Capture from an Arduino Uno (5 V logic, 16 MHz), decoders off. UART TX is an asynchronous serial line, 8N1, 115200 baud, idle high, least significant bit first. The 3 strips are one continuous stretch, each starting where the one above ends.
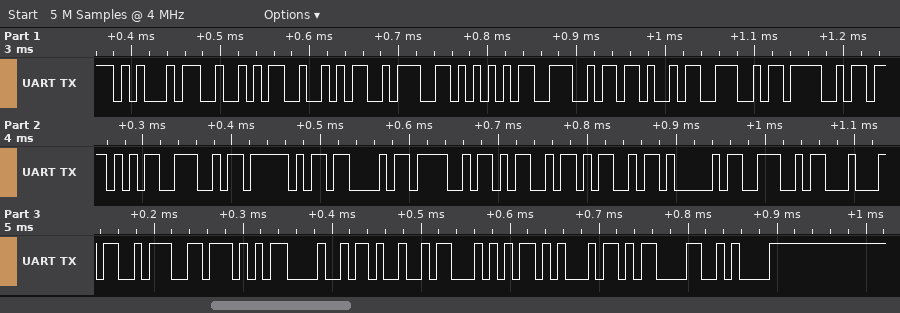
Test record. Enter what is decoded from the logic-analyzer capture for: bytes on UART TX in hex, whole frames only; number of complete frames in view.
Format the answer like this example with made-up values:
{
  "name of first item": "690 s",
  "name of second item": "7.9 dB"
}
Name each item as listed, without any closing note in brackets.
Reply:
{
  "bytes on UART TX in hex, whole frames only": "45 52 52 3A 55 4E 4B 4E 4F 57 4E 5F 43 4F 4D 4D 41 4E 44 3A 57 48 49 54 45 0D 0A",
  "number of complete frames in view": "27"
}
